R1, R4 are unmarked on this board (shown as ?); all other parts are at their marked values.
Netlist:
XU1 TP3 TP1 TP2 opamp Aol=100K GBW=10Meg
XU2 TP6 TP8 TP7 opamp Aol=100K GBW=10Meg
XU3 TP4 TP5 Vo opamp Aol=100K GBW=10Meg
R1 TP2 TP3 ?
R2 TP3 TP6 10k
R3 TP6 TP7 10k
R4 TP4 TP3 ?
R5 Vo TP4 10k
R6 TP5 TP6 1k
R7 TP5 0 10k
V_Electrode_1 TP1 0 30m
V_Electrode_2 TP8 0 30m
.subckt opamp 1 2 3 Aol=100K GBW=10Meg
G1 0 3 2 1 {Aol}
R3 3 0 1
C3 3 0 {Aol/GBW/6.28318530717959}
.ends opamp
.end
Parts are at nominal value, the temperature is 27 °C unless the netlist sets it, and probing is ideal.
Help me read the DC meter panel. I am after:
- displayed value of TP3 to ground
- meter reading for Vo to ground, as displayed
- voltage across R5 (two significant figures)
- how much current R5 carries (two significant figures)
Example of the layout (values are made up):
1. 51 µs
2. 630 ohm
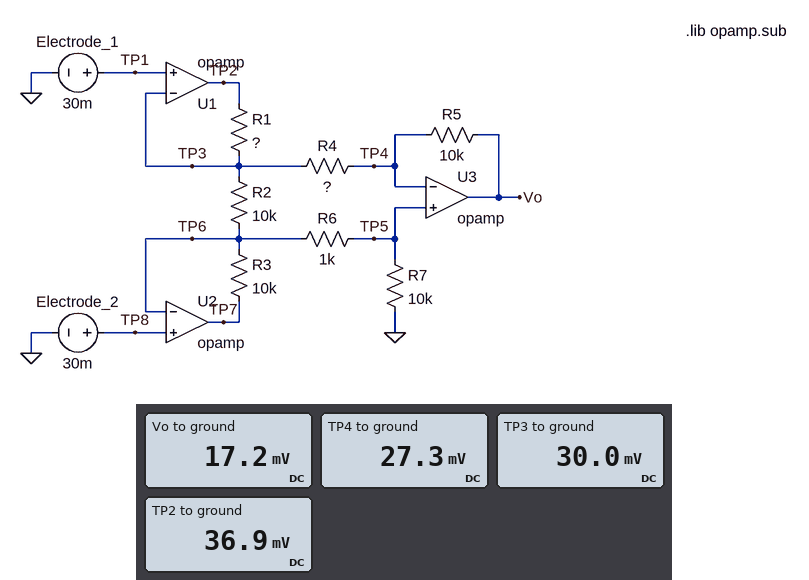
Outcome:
1. 30.0 mV
2. 17.2 mV
3. 10 mV
4. 1.0 µA
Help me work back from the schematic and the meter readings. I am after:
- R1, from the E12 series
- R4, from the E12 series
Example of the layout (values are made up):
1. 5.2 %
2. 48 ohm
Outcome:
1. 6.8 kΩ
2. 2.7 kΩ
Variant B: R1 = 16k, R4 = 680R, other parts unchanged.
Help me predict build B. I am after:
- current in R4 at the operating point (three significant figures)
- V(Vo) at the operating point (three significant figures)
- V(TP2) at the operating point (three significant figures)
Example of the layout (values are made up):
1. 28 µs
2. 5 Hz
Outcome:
1. 4.01 µA
2. -12.8 mV
3. 94.2 mV
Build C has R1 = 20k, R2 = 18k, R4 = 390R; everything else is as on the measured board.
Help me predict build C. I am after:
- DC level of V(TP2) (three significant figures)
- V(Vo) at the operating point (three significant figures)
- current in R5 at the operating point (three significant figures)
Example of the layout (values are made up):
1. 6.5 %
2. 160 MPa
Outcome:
1. 170 mV
2. -42.6 mV
3. 6.99 µA
